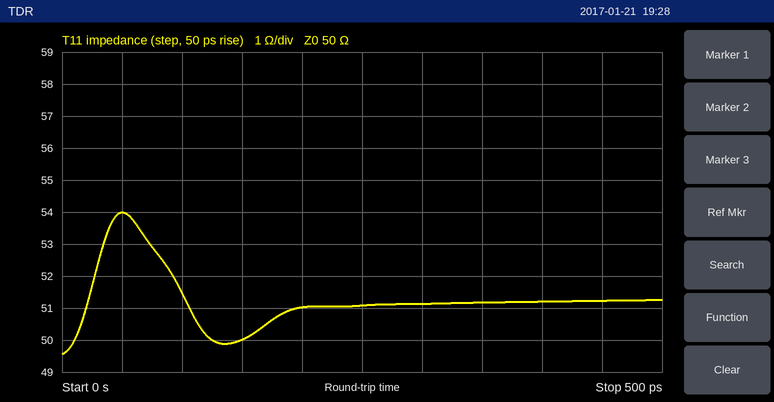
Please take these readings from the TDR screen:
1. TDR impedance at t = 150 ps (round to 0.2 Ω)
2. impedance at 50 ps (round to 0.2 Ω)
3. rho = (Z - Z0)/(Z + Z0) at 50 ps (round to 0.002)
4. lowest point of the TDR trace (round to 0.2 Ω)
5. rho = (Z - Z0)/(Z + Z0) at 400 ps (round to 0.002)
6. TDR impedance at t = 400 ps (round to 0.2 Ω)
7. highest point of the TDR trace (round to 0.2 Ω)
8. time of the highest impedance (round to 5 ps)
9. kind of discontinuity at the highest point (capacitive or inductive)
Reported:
50.0 Ω
54.0 Ω
+0.038
49.6 Ω
+0.012
51.2 Ω
54.0 Ω
50 ps
inductive
